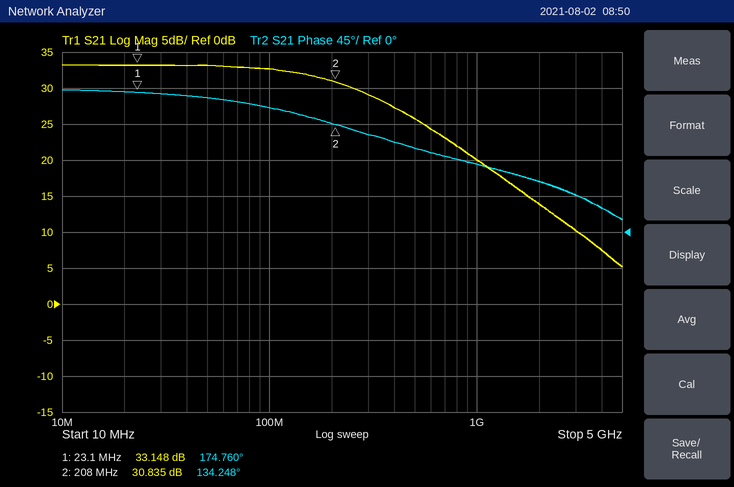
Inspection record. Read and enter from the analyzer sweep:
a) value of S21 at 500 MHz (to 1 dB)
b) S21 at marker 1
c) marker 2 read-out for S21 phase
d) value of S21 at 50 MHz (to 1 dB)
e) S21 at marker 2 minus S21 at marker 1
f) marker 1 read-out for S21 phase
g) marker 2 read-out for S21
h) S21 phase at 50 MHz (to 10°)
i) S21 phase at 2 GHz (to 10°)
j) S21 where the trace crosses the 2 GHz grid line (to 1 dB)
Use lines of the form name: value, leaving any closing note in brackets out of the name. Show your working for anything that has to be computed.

value of S21 at 500 MHz: 26 dB
S21 at marker 1: 33.148 dB
marker 2 read-out for S21 phase: 134.248°
value of S21 at 50 MHz: 33 dB
S21 at marker 2 minus S21 at marker 1: 30.835 − (33.148) = -2.313 dB
marker 1 read-out for S21 phase: 174.760°
marker 2 read-out for S21: 30.835 dB
S21 phase at 50 MHz: 170°
S21 phase at 2 GHz: 60°
S21 where the trace crosses the 2 GHz grid line: 14 dB
